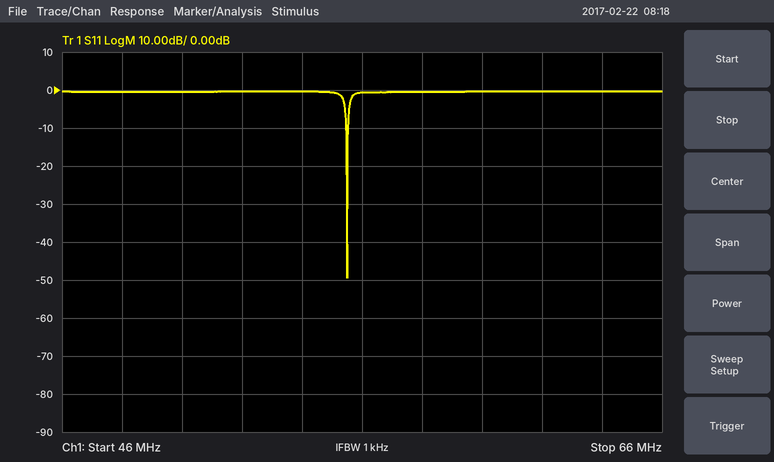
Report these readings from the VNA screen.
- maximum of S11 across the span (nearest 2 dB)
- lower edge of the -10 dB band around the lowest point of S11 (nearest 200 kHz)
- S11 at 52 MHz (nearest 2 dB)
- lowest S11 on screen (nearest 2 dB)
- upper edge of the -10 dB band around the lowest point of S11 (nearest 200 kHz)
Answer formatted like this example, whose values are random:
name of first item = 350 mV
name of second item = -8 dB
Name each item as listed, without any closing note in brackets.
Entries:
maximum of S11 across the span = 0 dB
lower edge of the -10 dB band around the lowest point of S11 = 55.4 MHz
S11 at 52 MHz = 0 dB
lowest S11 on screen = -50 dB
upper edge of the -10 dB band around the lowest point of S11 = 55.6 MHz
